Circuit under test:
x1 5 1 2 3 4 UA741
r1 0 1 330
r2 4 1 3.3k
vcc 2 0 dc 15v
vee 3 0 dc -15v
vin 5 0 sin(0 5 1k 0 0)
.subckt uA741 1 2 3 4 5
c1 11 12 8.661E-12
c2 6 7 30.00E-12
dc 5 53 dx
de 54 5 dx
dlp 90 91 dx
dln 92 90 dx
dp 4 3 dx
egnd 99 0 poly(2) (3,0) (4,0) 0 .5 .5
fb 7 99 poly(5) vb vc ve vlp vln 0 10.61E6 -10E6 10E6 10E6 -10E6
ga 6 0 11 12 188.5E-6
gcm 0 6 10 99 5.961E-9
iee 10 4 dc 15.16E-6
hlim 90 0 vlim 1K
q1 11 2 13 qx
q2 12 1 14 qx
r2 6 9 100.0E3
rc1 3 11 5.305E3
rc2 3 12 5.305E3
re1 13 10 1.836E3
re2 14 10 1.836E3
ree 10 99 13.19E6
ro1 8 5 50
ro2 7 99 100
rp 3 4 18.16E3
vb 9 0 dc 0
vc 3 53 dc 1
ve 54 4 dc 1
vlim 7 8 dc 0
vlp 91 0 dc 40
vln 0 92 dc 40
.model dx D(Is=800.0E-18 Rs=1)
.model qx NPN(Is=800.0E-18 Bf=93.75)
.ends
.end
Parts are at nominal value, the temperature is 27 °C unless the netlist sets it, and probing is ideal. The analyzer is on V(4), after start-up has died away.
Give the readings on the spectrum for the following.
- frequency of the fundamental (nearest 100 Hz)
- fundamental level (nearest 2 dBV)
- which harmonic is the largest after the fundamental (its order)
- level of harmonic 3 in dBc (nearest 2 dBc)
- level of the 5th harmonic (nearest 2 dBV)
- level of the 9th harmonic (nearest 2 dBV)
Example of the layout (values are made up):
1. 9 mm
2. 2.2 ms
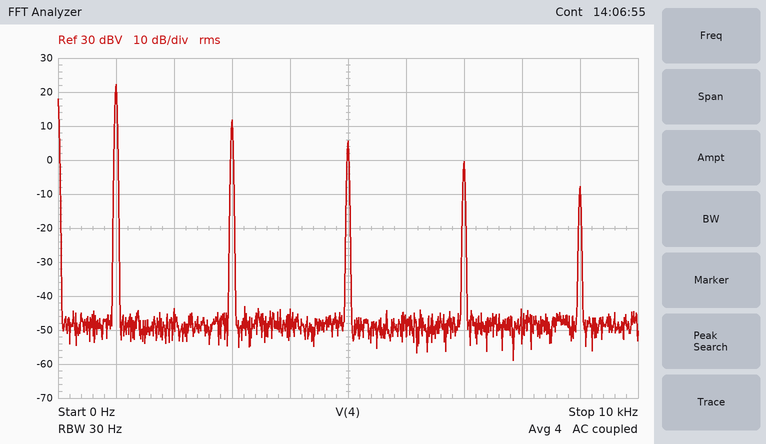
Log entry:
1. 1.0 kHz
2. 22 dBV
3. 3
4. -10 dBc
5. 6 dBV
6. -8 dBV
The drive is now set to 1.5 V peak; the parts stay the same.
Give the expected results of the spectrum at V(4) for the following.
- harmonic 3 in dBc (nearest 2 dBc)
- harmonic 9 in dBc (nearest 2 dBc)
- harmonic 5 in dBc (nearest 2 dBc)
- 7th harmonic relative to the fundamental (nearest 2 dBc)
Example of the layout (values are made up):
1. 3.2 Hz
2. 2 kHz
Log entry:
1. -28 dBc
2. -60 dBc
3. -32 dBc
4. -38 dBc
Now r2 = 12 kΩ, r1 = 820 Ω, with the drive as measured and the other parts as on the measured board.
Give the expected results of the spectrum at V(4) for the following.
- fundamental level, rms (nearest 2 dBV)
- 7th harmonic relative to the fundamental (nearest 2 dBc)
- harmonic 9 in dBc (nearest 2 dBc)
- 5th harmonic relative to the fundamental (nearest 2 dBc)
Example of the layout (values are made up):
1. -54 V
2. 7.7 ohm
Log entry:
1. 22 dBV
2. -20 dBc
3. -24 dBc
4. -16 dBc
